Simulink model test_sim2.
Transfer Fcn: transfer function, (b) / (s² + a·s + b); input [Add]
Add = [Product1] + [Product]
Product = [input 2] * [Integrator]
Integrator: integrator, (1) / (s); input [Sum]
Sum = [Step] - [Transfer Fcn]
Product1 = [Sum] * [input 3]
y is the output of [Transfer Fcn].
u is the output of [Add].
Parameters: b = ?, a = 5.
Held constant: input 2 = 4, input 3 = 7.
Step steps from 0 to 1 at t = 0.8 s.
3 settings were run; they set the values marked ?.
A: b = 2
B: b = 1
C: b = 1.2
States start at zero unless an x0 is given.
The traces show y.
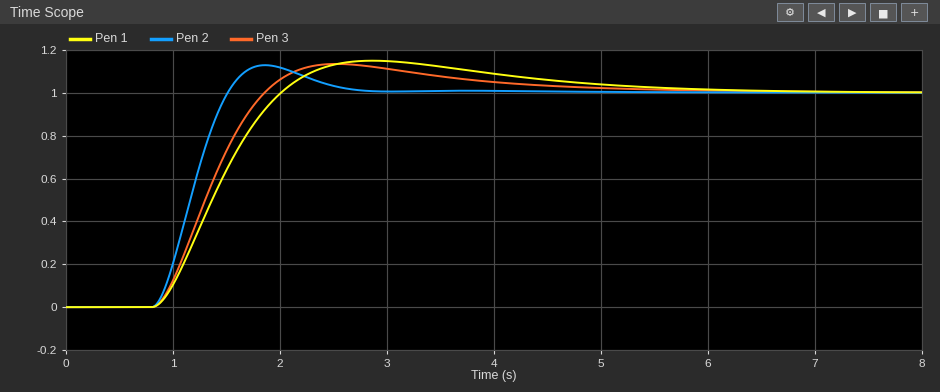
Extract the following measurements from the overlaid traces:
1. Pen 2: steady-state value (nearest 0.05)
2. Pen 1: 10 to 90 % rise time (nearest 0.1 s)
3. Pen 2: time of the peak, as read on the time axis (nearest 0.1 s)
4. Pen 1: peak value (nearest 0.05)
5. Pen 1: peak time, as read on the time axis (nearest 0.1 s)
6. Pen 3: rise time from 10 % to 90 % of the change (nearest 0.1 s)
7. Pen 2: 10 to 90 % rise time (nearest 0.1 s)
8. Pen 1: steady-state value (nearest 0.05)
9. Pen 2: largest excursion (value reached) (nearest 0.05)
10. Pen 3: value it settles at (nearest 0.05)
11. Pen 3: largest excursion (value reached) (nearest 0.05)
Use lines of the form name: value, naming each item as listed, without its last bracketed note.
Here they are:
Pen 2: steady-state value: 1.00
Pen 1: 10 to 90 % rise time: 0.8 s
Pen 2: time of the peak, as read on the time axis: 1.9 s
Pen 1: peak value: 1.15
Pen 1: peak time, as read on the time axis: 2.9 s
Pen 3: rise time from 10 % to 90 % of the change: 0.7 s
Pen 2: 10 to 90 % rise time: 0.5 s
Pen 1: steady-state value: 1.00
Pen 2: largest excursion (value reached): 1.15
Pen 3: value it settles at: 1.00
Pen 3: largest excursion (value reached): 1.15
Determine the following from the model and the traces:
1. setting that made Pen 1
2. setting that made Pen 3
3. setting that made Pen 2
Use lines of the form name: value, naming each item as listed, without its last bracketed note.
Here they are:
setting that made Pen 1: B
setting that made Pen 3: C
setting that made Pen 2: A
